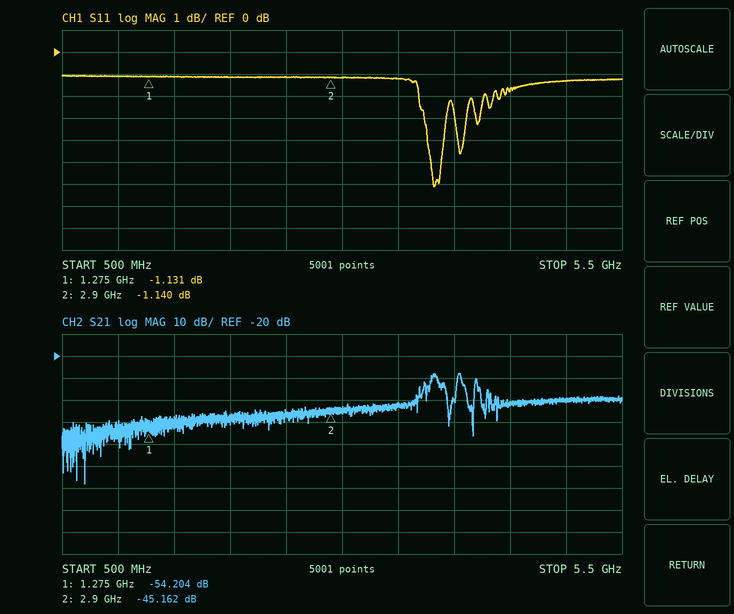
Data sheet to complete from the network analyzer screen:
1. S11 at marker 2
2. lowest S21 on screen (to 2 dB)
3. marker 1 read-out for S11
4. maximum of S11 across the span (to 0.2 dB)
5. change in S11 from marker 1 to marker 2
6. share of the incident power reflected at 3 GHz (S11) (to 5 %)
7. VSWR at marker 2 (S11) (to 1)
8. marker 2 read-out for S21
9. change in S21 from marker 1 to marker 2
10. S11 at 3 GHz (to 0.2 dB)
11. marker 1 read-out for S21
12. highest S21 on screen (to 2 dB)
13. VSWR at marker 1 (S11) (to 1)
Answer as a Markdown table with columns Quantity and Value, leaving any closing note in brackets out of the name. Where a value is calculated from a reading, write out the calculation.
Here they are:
| Quantity | Value |
|---|---|
| S11 at marker 2 | -1.140 dB |
| lowest S21 on screen | -78 dB |
| marker 1 read-out for S11 | -1.131 dB |
| maximum of S11 across the span | -1.0 dB |
| change in S11 from marker 1 to marker 2 | -1.14 − (-1.131) = -0.009 dB |
| share of the incident power reflected at 3 GHz (S11) | 10^(-1.2/10) ≈ 75.9 %, so 75 % to the nearest 5 % |
| VSWR at marker 2 (S11) | (1 + 0.8770)/(1 − 0.8770) ≈ 15 |
| marker 2 read-out for S21 | -45.162 dB |
| change in S21 from marker 1 to marker 2 | -45.162 − (-54.204) = 9.042 dB |
| S11 at 3 GHz | -1.2 dB |
| marker 1 read-out for S21 | -54.204 dB |
| highest S21 on screen | -28 dB |
| VSWR at marker 1 (S11) | (1 + 0.8779)/(1 − 0.8779) ≈ 15 |
